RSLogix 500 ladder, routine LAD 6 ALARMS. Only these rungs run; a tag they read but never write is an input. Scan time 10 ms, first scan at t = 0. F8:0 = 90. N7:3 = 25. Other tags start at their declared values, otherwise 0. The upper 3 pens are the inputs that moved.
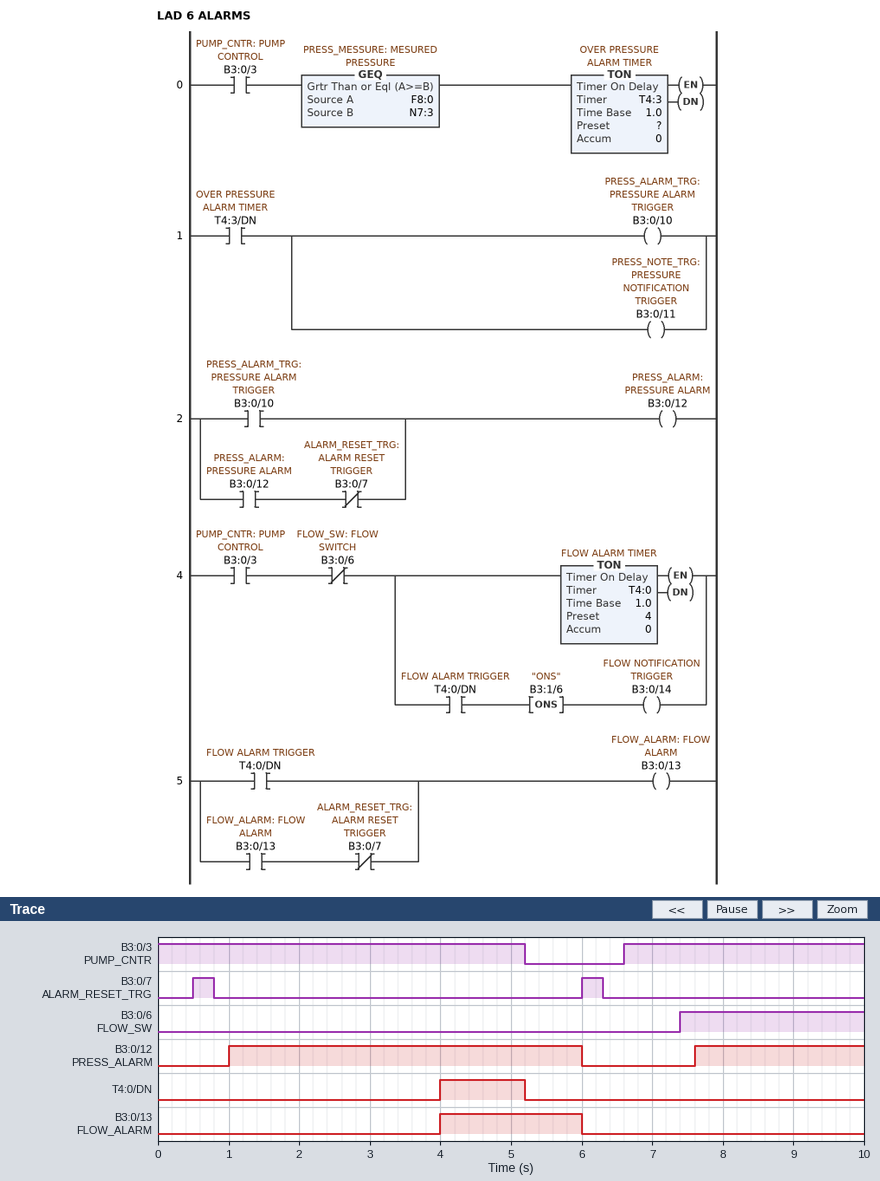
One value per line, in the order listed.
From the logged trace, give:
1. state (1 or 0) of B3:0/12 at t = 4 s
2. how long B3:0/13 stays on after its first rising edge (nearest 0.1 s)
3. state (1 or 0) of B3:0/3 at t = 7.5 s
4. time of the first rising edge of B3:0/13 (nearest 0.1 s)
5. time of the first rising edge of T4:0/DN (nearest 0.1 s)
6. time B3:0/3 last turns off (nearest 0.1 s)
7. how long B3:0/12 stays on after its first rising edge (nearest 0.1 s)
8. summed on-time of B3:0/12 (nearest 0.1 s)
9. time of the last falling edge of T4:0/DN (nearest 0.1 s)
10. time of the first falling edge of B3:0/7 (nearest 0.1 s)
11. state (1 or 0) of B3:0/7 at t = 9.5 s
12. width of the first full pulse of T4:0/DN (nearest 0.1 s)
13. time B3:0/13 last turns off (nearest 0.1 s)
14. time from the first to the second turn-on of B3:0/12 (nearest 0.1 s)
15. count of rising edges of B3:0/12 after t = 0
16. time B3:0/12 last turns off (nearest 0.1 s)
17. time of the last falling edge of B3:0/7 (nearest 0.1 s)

1
2.0 s
1
4.0 s
4.0 s
5.2 s
5.0 s
7.4 s
5.2 s
0.8 s
0
1.2 s
6.0 s
6.6 s
2
6.0 s
6.3 s
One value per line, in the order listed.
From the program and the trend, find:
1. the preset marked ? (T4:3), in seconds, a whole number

1 s
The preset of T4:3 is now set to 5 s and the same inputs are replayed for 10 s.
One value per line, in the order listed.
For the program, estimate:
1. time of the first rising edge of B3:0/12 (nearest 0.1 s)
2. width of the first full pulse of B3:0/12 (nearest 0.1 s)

5.0 s
1.0 s
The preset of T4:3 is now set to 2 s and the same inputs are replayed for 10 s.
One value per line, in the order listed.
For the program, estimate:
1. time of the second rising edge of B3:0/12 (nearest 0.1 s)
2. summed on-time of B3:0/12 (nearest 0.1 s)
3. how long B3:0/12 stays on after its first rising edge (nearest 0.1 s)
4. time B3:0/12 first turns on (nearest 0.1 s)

8.6 s
5.4 s
4.0 s
2.0 s
